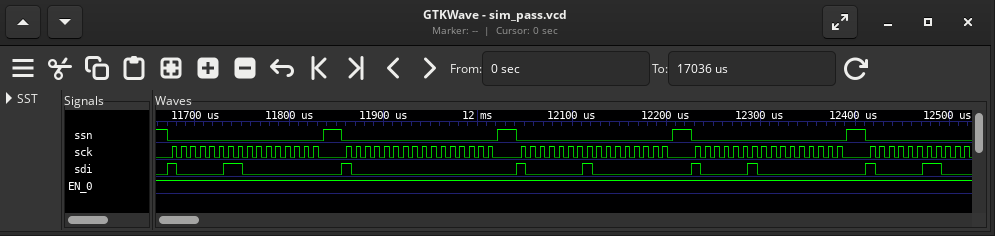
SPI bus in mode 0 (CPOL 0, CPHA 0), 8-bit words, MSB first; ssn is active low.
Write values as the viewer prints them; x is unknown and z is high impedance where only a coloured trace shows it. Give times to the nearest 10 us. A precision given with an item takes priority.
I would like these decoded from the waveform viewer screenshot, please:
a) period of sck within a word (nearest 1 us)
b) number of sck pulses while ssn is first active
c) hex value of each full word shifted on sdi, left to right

10 us
16
83, 00, 80, 00, 81, 00, 82, 00, 83
